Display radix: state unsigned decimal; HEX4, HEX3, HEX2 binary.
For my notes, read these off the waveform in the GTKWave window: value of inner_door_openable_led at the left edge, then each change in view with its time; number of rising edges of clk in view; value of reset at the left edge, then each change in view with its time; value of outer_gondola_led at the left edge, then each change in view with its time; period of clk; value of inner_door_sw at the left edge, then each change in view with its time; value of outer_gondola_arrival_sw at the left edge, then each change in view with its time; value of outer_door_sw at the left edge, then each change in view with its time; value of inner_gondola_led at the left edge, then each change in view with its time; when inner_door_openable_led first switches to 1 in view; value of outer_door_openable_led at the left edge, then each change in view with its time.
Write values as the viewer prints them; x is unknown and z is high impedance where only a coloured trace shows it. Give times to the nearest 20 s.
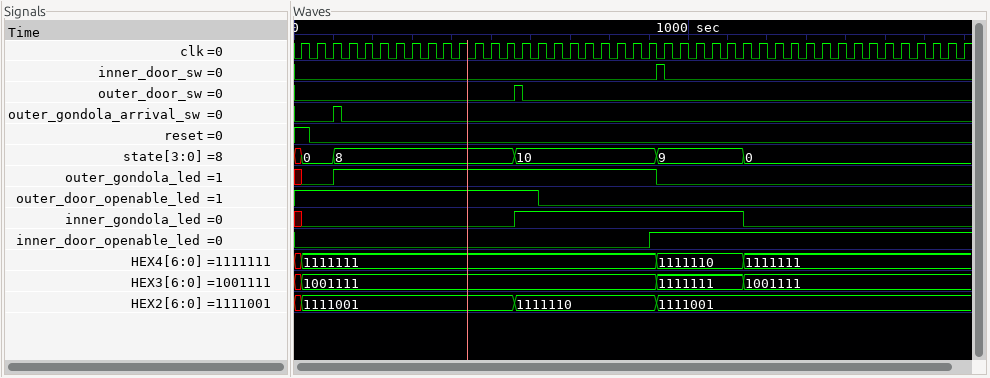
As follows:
0, 1 at 900 s
43
1, 0 at 40 s
x, 0 at 20 s, 1 at 100 s, 0 at 920 s
40 s
0, 1 at 920 s, 0 at 940 s
0, 1 at 100 s, 0 at 120 s
0, 1 at 560 s, 0 at 580 s
x, 0 at 20 s, 1 at 560 s, 0 at 1140 s
900 s
1, 0 at 620 s
